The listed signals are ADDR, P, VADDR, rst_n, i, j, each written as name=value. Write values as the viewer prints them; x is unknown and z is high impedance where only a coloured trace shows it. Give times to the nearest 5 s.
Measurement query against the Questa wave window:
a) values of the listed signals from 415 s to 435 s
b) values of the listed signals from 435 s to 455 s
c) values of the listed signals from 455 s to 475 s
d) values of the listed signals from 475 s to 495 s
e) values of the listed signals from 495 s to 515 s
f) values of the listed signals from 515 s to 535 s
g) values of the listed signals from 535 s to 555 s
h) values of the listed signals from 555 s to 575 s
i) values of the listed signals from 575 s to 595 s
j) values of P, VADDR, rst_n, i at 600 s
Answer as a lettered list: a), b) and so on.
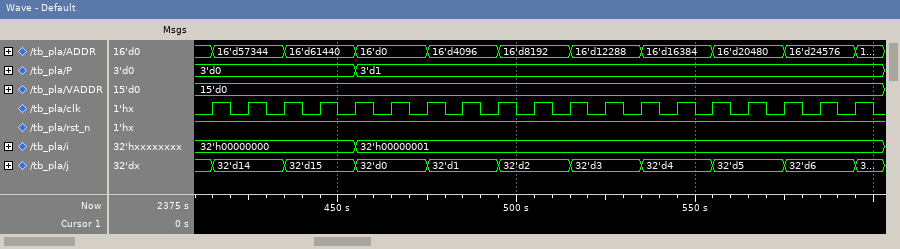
a) ADDR=16'd57344, P=3'd0, VADDR=15'd0, rst_n=1, i=32'h00000000, j=32'd14
b) ADDR=16'd61440, P=3'd0, VADDR=15'd0, rst_n=1, i=32'h00000000, j=32'd15
c) ADDR=16'd0, P=3'd1, VADDR=15'd0, rst_n=1, i=32'h00000001, j=32'd0
d) ADDR=16'd4096, P=3'd1, VADDR=15'd0, rst_n=1, i=32'h00000001, j=32'd1
e) ADDR=16'd8192, P=3'd1, VADDR=15'd0, rst_n=1, i=32'h00000001, j=32'd2
f) ADDR=16'd12288, P=3'd1, VADDR=15'd0, rst_n=1, i=32'h00000001, j=32'd3
g) ADDR=16'd16384, P=3'd1, VADDR=15'd0, rst_n=1, i=32'h00000001, j=32'd4
h) ADDR=16'd20480, P=3'd1, VADDR=15'd0, rst_n=1, i=32'h00000001, j=32'd5
i) ADDR=16'd24576, P=3'd1, VADDR=15'd0, rst_n=1, i=32'h00000001, j=32'd6
j) P=3'd1, VADDR=15'd0, rst_n=1, i=32'h00000001
